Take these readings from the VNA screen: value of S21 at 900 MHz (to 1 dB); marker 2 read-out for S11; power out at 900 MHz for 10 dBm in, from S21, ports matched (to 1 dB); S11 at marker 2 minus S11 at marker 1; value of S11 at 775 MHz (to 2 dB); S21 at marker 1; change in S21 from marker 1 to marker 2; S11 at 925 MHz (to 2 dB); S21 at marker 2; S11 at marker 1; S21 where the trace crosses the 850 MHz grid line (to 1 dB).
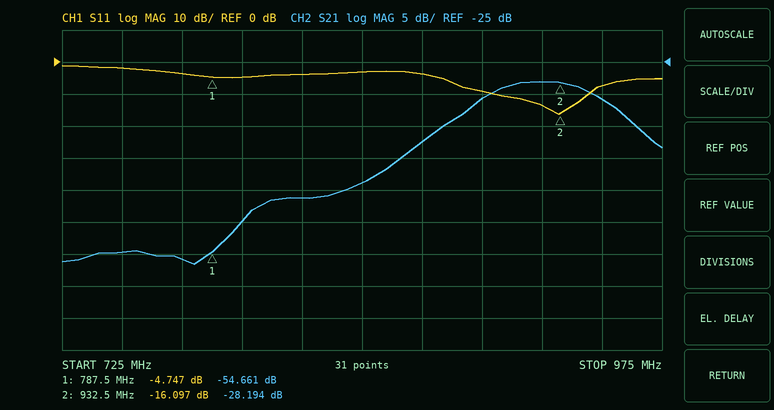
-31 dB
-16.097 dB
-21 dBm
-11.350 dB
-4 dB
-54.661 dB
26.467 dB
-14 dB
-28.194 dB
-4.747 dB
-44 dB
